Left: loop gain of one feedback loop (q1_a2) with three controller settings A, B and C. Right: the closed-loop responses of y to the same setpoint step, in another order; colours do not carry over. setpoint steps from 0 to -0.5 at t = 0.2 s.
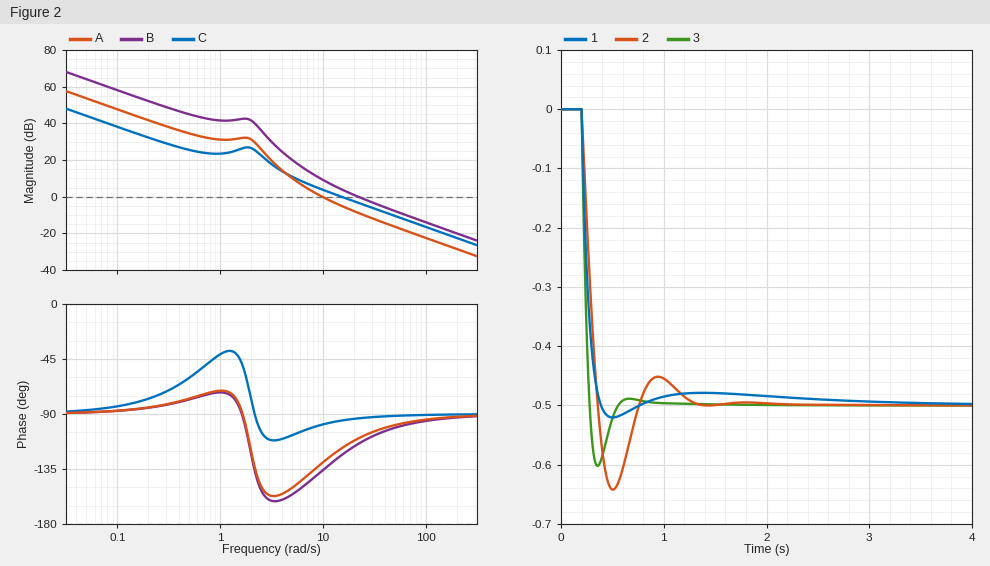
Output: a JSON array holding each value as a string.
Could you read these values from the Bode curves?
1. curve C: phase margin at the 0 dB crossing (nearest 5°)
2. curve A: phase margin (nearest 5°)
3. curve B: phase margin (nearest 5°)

["85°", "50°", "65°"]
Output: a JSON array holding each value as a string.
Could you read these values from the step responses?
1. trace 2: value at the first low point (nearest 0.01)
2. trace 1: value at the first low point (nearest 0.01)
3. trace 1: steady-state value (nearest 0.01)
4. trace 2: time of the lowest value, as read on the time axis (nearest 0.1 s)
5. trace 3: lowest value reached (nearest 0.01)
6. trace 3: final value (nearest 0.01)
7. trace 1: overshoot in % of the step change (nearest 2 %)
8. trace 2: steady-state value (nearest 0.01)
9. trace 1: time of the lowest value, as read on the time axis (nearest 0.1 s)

["-0.64", "-0.52", "-0.50", "0.5 s", "-0.60", "-0.50", "4 %", "-0.50", "0.5 s"]
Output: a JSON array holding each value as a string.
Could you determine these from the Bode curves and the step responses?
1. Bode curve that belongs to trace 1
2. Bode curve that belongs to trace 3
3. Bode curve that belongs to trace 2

["C", "B", "A"]
